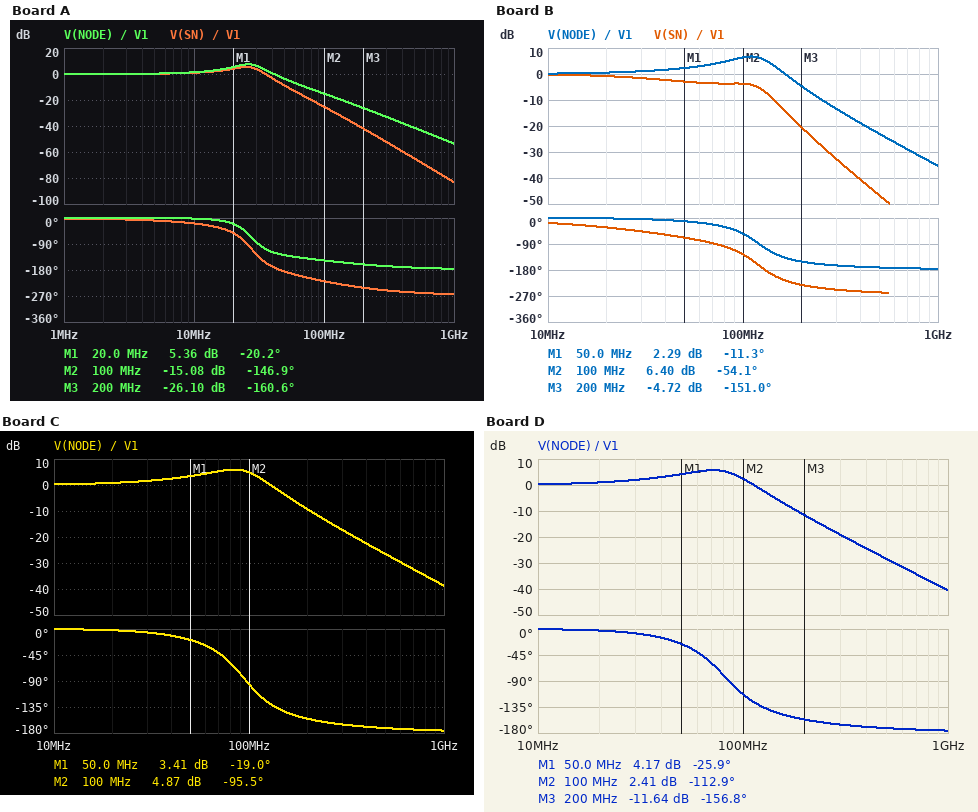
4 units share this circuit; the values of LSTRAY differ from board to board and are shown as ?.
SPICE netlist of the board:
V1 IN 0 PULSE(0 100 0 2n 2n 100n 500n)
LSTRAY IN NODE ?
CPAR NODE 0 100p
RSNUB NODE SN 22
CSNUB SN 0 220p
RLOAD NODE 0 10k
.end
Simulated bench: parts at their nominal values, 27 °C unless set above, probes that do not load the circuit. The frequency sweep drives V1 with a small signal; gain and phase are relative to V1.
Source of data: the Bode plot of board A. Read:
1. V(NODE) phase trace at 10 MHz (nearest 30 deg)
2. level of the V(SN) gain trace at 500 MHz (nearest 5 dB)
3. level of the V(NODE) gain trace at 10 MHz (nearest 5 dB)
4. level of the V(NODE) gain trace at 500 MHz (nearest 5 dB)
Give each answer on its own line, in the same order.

0 deg
-65 dB
0 dB
-40 dB
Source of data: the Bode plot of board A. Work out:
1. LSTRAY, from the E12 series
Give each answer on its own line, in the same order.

120 nH
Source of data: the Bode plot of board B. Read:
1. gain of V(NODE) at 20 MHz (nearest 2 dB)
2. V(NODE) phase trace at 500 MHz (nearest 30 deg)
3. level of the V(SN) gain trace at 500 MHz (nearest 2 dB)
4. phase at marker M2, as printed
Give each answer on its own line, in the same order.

0 dB
-180 deg
-46 dB
-54.1 deg
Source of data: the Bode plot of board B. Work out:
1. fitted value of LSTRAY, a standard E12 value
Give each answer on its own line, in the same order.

15 nH
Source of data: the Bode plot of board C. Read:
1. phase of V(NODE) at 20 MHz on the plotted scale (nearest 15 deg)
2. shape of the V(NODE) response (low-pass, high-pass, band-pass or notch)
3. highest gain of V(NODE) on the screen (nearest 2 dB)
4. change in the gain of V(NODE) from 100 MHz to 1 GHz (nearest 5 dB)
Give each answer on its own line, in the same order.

0 deg
low-pass
6 dB
-45 dB
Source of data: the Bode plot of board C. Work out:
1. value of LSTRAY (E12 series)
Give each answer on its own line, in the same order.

22 nH
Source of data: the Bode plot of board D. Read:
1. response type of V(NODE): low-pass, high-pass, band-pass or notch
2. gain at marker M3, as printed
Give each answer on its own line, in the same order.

low-pass
-11.64 dB
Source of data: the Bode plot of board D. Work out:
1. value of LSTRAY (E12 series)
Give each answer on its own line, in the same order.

27 nH
